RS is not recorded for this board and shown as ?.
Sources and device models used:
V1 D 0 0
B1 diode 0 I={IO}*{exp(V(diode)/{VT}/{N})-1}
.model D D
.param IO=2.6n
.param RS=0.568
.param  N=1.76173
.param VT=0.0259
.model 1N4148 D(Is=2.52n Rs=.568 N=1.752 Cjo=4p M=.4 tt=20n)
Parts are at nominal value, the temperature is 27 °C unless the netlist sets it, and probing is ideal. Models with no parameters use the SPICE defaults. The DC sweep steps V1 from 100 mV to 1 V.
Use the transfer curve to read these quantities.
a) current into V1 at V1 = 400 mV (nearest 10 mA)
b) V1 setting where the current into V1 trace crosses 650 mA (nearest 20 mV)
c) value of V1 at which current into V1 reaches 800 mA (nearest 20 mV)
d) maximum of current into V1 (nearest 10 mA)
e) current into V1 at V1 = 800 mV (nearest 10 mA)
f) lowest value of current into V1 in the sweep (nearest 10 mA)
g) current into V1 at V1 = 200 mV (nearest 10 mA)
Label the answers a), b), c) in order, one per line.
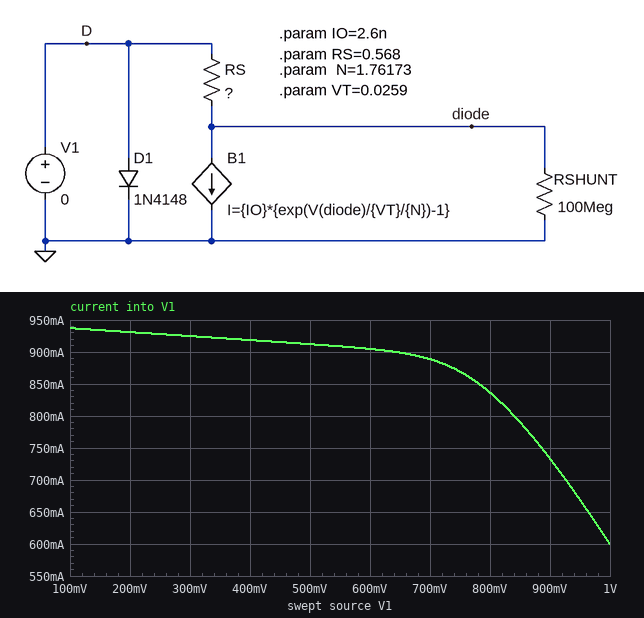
a) 920 mA
b) 960 mV
c) 840 mV
d) 940 mA
e) 840 mA
f) 600 mA
g) 930 mA
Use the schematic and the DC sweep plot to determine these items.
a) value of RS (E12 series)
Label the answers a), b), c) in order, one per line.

a) 1.5 Ω
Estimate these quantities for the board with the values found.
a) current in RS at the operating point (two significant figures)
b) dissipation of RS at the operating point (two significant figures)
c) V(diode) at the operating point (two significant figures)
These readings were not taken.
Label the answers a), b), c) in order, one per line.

a) 940 mA
b) 1.3 W
c) 1.4 V
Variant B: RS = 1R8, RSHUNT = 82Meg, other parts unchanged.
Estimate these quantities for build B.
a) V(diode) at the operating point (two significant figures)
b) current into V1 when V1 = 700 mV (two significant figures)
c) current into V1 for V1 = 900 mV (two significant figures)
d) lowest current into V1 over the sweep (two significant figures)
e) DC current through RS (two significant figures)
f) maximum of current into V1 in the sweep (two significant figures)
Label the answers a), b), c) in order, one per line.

a) 1.7 V
b) 870 mA
c) 720 mA
d) 580 mA
e) 930 mA
f) 920 mA
